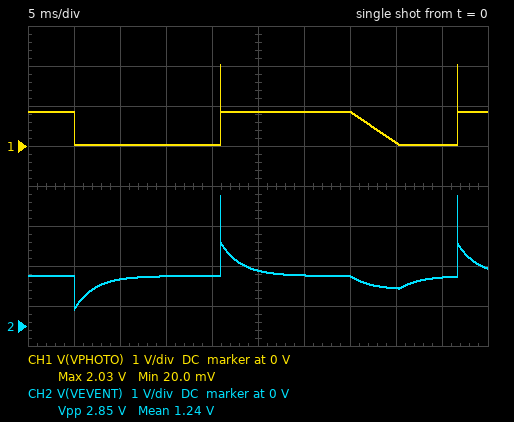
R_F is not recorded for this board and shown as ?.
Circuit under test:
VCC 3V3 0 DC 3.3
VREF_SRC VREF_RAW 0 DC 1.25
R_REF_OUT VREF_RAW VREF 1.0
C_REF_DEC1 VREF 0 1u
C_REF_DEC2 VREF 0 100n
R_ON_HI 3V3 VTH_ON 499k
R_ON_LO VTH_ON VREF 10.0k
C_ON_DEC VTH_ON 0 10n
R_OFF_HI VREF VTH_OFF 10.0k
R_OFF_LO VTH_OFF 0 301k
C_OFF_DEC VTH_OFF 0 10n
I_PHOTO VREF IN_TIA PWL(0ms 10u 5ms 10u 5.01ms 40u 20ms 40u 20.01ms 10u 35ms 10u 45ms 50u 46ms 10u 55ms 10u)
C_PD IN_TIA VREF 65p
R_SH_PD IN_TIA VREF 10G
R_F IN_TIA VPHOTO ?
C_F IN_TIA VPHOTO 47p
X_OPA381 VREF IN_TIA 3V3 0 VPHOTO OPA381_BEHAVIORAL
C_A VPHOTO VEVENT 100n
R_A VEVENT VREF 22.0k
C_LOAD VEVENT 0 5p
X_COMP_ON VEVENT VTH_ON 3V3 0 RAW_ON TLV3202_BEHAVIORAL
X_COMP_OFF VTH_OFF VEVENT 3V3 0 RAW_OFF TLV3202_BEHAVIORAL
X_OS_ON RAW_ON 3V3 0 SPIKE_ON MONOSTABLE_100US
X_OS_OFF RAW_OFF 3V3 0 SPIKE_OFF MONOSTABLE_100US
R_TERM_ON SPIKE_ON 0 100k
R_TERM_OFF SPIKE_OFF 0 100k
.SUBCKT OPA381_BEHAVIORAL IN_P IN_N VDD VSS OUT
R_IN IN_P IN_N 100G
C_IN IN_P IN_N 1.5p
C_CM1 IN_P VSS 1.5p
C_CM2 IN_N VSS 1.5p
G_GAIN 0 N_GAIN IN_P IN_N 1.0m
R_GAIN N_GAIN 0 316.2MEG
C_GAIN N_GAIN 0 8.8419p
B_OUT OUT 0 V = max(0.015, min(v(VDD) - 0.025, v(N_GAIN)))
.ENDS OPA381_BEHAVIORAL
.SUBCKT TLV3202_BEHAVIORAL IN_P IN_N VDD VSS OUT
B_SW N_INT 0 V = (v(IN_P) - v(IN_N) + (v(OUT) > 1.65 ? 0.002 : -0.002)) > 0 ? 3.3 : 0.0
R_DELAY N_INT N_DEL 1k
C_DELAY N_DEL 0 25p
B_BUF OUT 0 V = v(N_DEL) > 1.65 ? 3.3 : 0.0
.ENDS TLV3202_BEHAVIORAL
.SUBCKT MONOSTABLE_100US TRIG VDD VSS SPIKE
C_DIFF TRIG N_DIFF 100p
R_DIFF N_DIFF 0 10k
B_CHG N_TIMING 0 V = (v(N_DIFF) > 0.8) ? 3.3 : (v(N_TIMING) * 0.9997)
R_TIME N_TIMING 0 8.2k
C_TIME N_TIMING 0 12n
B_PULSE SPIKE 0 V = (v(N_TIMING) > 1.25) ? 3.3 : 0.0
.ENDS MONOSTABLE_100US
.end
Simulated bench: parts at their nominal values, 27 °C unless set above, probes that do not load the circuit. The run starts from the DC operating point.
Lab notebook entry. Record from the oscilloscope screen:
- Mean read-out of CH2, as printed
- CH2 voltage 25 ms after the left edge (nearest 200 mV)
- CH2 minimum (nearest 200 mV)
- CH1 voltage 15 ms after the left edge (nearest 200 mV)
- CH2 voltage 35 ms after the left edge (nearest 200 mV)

1.24 V
1.4 V
400 mV
0 V
1.2 V
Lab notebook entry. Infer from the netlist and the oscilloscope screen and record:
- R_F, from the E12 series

39 kΩ
